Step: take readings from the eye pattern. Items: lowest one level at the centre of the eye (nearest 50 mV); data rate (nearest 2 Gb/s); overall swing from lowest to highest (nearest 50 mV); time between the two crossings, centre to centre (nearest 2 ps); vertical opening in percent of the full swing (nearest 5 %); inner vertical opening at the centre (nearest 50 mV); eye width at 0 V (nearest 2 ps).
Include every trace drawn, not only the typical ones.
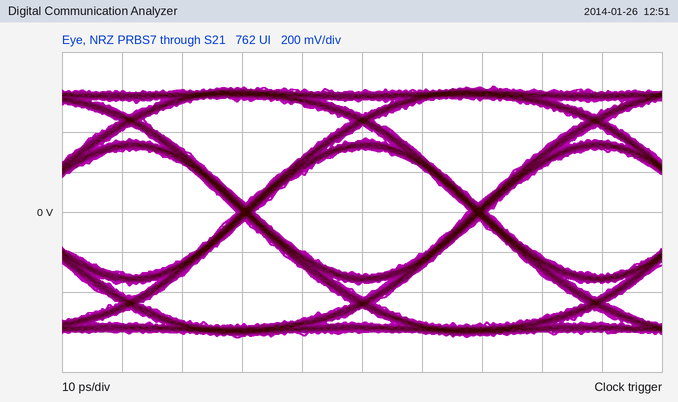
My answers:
300 mV
26 Gb/s
1.25 V
38 ps
50 %
650 mV
36 ps
